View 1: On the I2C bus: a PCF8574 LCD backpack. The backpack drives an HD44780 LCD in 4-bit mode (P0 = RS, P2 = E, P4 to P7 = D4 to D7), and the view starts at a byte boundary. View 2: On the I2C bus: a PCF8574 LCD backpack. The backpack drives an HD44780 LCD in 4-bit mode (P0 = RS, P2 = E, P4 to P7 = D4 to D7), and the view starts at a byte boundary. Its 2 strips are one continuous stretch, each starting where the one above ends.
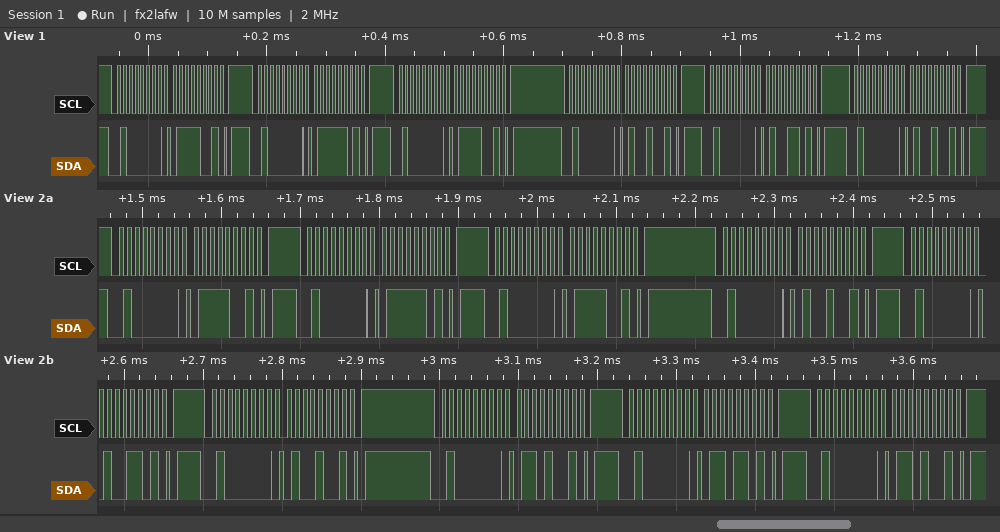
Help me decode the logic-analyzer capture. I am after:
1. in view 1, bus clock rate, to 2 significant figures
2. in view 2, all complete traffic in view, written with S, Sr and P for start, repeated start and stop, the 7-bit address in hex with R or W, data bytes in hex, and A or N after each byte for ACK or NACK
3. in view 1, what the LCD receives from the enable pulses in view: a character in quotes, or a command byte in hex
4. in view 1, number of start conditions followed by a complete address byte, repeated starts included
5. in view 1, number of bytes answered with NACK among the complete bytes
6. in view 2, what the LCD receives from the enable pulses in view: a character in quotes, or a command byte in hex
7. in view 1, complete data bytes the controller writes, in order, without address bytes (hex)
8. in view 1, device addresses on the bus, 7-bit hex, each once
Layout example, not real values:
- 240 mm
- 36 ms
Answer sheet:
- 100 kHz
- S 20W A 79 A P S 20W A 7D A P S 20W A 79 A P S 20W A 49 A P S 20W A 4D A P S 20W A 49 A P S 20W A 69 A P S 20W A 6D A P S 20W A 69 A P
- 't'
- 6
- 0
- 't'
- 79 7D 79 49 4D 49
- 0x20
